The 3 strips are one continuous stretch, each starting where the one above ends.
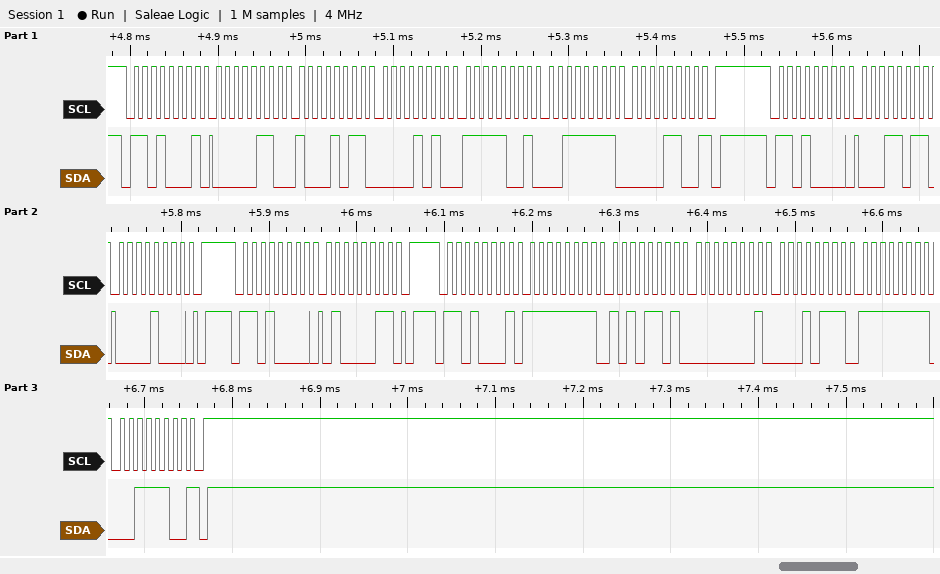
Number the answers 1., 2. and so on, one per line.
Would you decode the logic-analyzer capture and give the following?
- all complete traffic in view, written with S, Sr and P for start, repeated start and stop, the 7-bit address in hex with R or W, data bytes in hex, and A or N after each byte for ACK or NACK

1. S 68R A 06 A 8B A 0A A F9 A 3F A 0C N P S 68W A 1B A 08 A P S 68W A 43 A P S 68R A FF A AD A 01 A 17 A FF A 3C N P
